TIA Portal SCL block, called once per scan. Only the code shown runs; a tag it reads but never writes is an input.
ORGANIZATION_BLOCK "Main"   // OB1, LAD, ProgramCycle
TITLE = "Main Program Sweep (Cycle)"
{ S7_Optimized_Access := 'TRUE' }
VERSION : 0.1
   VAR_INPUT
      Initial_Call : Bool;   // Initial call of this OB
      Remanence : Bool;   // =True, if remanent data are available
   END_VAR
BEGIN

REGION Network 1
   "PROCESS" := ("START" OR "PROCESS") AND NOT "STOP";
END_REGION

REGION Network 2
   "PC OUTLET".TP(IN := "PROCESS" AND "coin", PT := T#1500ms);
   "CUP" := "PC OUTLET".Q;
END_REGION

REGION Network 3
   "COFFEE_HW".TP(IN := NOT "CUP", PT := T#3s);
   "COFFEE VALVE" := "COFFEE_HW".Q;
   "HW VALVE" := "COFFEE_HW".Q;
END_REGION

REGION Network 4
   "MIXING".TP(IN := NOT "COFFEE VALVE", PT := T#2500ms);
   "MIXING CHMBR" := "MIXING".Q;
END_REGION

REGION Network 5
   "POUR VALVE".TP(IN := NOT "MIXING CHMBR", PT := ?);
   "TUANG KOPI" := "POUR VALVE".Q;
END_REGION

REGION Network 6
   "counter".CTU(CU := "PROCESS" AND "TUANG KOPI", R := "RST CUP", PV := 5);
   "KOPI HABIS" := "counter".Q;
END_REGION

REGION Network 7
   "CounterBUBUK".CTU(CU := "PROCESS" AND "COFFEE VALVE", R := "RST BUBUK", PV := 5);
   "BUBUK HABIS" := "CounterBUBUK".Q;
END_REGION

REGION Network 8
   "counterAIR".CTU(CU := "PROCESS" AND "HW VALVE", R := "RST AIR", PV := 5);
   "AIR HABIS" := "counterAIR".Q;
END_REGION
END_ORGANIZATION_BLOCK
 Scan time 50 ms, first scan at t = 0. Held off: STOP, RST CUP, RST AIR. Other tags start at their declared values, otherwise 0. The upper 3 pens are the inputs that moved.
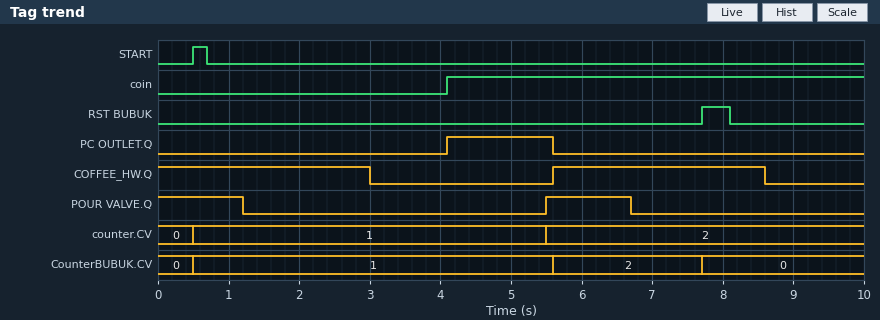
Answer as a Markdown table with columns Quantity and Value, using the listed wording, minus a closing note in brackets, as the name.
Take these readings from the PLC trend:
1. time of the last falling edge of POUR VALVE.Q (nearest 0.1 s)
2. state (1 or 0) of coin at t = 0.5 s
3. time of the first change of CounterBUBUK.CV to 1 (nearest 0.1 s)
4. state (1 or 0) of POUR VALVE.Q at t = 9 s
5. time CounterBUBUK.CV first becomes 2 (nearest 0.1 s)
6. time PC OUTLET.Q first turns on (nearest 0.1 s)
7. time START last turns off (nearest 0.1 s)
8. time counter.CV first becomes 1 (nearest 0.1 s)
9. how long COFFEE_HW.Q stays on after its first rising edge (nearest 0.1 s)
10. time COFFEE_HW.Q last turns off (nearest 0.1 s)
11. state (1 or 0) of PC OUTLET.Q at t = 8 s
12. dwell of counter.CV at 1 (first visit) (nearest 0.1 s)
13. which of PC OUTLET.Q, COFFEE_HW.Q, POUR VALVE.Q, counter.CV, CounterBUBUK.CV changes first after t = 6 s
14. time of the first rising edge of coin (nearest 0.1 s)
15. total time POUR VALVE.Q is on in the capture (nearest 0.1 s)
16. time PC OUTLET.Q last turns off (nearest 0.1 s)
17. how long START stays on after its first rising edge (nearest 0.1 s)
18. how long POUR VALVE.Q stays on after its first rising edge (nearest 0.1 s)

| Quantity | Value |
|---|---|
| time of the last falling edge of POUR VALVE.Q | 6.7 s |
| state (1 or 0) of coin at t = 0.5 s | 0 |
| time of the first change of CounterBUBUK.CV to 1 | 0.5 s |
| state (1 or 0) of POUR VALVE.Q at t = 9 s | 0 |
| time CounterBUBUK.CV first becomes 2 | 5.6 s |
| time PC OUTLET.Q first turns on | 4.1 s |
| time START last turns off | 0.7 s |
| time counter.CV first becomes 1 | 0.5 s |
| how long COFFEE_HW.Q stays on after its first rising edge | 3.0 s |
| time COFFEE_HW.Q last turns off | 8.6 s |
| state (1 or 0) of PC OUTLET.Q at t = 8 s | 0 |
| dwell of counter.CV at 1 (first visit) | 5.0 s |
| which of PC OUTLET.Q, COFFEE_HW.Q, POUR VALVE.Q, counter.CV, CounterBUBUK.CV changes first after t = 6 s | POUR VALVE.Q |
| time of the first rising edge of coin | 4.1 s |
| total time POUR VALVE.Q is on in the capture | 2.4 s |
| time PC OUTLET.Q last turns off | 5.6 s |
| how long START stays on after its first rising edge | 0.2 s |
| how long POUR VALVE.Q stays on after its first rising edge | 1.2 s |
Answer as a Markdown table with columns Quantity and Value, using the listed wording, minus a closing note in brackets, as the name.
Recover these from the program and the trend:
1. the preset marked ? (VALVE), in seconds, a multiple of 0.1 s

| Quantity | Value |
|---|---|
| the preset marked ? (VALVE), in seconds, a multiple of 0.1 s | 1.2 s |
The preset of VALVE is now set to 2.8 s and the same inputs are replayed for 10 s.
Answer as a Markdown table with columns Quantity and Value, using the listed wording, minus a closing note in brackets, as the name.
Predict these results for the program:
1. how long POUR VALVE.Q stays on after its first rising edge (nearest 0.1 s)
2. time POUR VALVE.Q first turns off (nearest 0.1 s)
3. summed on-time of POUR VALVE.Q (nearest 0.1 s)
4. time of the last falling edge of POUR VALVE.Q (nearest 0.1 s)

| Quantity | Value |
|---|---|
| how long POUR VALVE.Q stays on after its first rising edge | 2.8 s |
| time POUR VALVE.Q first turns off | 2.8 s |
| summed on-time of POUR VALVE.Q | 5.6 s |
| time of the last falling edge of POUR VALVE.Q | 8.3 s |
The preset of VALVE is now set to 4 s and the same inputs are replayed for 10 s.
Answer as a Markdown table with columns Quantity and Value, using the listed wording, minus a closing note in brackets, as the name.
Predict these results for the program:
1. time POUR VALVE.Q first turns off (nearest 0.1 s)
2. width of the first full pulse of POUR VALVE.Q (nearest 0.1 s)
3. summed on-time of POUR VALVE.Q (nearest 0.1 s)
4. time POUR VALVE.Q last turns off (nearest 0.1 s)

| Quantity | Value |
|---|---|
| time POUR VALVE.Q first turns off | 4.0 s |
| width of the first full pulse of POUR VALVE.Q | 4.0 s |
| summed on-time of POUR VALVE.Q | 8.0 s |
| time POUR VALVE.Q last turns off | 9.5 s |
